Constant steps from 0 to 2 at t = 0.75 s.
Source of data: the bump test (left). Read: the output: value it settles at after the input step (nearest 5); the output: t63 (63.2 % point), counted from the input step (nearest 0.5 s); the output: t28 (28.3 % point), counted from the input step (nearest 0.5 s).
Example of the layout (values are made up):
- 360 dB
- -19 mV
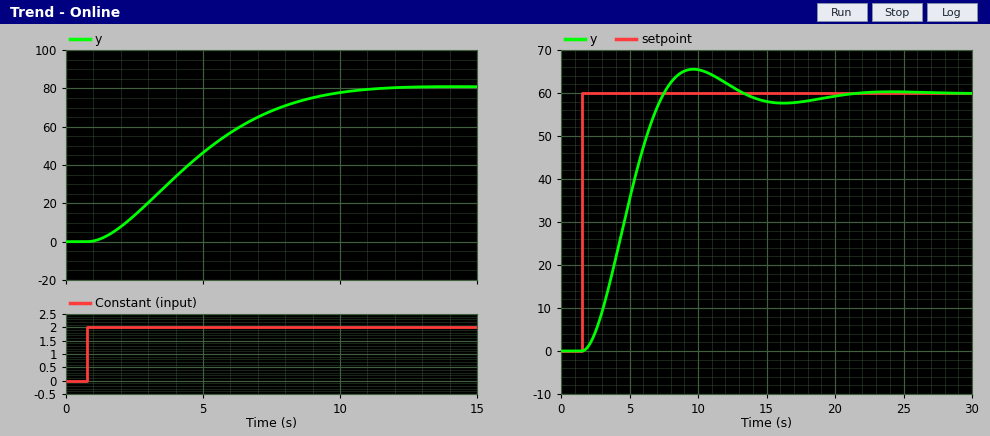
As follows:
- 80
- 4.5 s
- 2.5 s
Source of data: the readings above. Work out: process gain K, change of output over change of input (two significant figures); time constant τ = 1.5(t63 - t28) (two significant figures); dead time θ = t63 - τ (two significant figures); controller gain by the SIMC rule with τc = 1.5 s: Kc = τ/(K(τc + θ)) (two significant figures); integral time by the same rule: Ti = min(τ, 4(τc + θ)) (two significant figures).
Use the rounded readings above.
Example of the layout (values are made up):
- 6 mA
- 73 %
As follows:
- 40
- 3.0 s
- 1.5 s
- 0.025
- 3.0 s
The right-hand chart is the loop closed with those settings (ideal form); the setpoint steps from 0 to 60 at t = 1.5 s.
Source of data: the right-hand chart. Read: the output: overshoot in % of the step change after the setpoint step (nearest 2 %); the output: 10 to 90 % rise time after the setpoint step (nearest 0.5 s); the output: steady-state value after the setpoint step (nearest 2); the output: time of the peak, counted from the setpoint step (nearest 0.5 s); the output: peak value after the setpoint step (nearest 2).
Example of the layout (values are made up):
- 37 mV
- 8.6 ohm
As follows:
- 10 %
- 4.0 s
- 60
- 8.0 s
- 66
